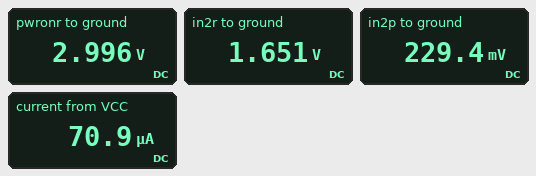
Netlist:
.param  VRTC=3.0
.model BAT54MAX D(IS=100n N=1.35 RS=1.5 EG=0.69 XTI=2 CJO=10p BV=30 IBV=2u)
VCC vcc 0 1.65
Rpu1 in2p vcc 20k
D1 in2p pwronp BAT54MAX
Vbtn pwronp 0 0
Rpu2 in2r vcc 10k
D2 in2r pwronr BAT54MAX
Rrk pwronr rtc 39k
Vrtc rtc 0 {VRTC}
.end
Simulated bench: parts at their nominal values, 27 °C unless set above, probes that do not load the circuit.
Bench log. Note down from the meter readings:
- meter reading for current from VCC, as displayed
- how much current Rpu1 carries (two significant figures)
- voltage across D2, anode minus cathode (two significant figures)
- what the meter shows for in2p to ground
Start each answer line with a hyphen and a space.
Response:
- 70.9 µA
- 71 µA
- -1.3 V
- 229.4 mV
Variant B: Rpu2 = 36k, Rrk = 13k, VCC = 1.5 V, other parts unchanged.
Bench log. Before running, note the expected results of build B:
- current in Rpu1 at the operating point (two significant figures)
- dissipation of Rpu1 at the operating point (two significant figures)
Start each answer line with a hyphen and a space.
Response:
- 64 µA
- 81 µW
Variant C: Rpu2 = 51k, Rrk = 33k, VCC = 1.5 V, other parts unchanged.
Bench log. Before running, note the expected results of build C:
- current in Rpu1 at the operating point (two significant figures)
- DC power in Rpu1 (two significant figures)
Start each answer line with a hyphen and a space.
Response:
- 64 µA
- 81 µW
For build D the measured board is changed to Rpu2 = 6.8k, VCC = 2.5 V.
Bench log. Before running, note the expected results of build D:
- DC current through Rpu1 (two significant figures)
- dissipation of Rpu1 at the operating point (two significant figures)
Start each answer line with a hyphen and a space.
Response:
- 110 µA
- 250 µW
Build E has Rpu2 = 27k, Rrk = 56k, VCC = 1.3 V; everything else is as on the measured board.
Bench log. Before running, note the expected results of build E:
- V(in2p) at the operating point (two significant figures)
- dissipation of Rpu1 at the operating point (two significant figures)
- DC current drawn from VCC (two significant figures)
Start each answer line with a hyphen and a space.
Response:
- 220 mV
- 58 µW
- 54 µA
